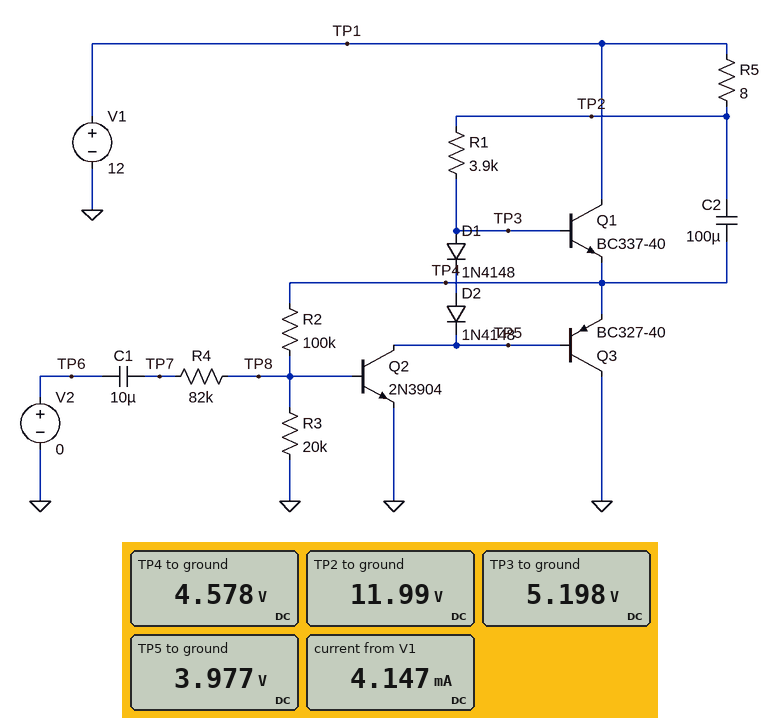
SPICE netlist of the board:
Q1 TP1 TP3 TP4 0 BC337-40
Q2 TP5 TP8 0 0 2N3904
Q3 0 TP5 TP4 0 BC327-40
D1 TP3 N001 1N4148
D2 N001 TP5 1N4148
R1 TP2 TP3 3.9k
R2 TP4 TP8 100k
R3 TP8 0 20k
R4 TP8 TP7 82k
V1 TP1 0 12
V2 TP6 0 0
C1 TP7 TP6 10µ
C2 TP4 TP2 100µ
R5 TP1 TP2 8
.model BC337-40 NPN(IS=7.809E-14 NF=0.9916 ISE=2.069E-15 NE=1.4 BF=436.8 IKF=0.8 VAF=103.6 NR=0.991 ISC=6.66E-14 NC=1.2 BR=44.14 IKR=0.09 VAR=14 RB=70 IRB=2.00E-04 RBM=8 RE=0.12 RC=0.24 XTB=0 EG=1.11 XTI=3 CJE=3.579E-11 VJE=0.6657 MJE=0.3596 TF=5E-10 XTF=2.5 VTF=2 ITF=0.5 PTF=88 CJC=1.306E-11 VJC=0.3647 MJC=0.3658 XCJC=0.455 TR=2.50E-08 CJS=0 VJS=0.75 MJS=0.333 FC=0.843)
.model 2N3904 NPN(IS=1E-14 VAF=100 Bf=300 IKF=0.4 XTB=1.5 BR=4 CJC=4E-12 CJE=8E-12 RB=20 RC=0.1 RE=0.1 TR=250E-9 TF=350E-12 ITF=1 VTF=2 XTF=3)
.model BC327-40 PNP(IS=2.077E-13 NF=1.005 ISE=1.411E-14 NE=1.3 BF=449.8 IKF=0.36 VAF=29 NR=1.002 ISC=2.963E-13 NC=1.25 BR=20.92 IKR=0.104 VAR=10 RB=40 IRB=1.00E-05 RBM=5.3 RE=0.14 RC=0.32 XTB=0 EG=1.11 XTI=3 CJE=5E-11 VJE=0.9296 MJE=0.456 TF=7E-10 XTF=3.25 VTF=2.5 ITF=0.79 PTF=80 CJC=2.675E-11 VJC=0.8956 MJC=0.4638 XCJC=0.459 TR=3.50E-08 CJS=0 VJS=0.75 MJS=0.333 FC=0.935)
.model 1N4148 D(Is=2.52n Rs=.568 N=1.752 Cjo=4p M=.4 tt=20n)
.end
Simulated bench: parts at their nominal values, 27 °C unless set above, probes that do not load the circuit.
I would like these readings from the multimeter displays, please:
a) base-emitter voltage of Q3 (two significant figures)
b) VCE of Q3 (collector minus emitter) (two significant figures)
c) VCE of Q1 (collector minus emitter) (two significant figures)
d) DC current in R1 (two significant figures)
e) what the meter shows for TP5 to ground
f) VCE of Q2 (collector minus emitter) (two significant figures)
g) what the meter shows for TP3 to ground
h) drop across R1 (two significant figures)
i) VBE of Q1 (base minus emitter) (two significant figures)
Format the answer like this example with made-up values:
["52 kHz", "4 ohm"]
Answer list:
["-600 mV", "-4.6 V", "7.4 V", "1.7 mA", "3.977 V", "4.0 V", "5.198 V", "6.8 V", "620 mV"]
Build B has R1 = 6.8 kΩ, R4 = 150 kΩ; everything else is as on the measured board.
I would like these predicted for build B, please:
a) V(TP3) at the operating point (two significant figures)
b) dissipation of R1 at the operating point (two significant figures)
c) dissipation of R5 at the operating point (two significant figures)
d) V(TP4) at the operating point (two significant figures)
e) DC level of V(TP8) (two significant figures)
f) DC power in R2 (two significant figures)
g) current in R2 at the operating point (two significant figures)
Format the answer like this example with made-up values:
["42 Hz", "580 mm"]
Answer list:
["4.9 V", "7.5 mW", "8.8 µW", "4.3 V", "660 mV", "130 µW", "36 µA"]
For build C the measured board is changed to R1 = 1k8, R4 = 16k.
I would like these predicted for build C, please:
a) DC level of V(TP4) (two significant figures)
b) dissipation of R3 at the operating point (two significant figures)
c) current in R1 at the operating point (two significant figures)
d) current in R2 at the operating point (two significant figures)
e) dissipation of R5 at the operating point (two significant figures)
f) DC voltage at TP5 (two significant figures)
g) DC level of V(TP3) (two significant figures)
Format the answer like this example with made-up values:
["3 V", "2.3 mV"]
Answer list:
["5.2 V", "24 µW", "3.4 mA", "45 µA", "92 µW", "4.6 V", "5.9 V"]
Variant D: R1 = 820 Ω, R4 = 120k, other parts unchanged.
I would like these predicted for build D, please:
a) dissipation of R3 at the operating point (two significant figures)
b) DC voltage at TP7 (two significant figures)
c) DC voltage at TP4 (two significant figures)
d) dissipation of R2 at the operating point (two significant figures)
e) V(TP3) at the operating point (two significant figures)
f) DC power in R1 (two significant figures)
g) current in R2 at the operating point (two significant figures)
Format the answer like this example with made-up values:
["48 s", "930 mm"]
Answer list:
["25 µW", "700 mV", "6.2 V", "300 µW", "6.9 V", "31 mW", "55 µA"]
